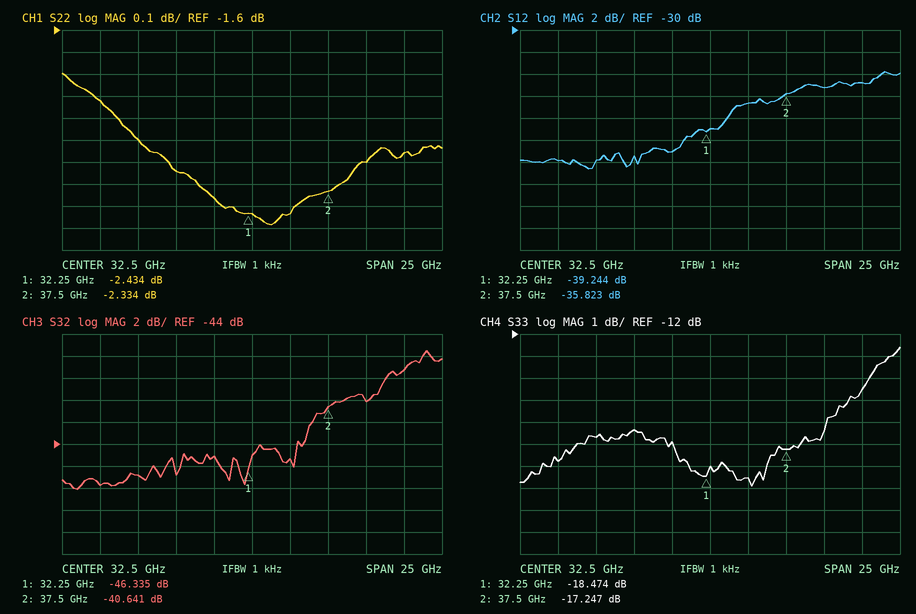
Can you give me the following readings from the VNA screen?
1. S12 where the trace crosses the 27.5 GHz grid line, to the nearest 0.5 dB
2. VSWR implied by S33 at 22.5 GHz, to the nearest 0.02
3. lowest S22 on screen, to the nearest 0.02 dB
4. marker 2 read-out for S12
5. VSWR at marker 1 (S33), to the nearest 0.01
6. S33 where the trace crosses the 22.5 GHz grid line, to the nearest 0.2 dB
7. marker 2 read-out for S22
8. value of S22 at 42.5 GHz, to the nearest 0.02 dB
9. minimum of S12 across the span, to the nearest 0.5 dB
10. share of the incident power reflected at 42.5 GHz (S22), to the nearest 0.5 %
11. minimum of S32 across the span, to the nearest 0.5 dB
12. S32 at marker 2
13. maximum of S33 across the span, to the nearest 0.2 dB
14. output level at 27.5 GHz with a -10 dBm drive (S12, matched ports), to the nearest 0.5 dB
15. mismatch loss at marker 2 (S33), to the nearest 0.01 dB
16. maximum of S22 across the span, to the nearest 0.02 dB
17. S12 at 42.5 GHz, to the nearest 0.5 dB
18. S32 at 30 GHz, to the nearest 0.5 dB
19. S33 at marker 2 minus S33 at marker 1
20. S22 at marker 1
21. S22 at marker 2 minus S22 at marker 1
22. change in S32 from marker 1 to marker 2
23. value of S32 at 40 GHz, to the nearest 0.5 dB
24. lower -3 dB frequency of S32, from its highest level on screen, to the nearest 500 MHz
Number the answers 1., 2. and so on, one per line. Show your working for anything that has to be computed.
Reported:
1. -41.5 dB
2. |Γ| = 10^(-17.8/20) = 0.1288; VSWR = (1 + 0.1288)/(1 − 0.1288) ≈ 1.30
3. -2.48 dB
4. -35.823 dB
5. (1 + 0.1192)/(1 − 0.1192) ≈ 1.27
6. -17.8 dB
7. -2.334 dB
8. -2.16 dB
9. -42.5 dB
10. 10^(-2.16/10) ≈ 60.8 %, so 61.0 % to the nearest 0.5 %
11. -48.0 dB
12. -40.641 dB
13. -12.6 dB
14. -10 dBm + (-41.5 dB) = -51.5 dBm
15. −10 log10(1 − 10^(-17.247/10)) ≈ 0.08 dB
16. -1.80 dB
17. -35.0 dB
18. -45.0 dB
19. -17.247 − (-18.474) = 1.227 dB
20. -2.434 dB
21. -2.334 − (-2.434) = 0.100 dB
22. -40.641 − (-46.335) = 5.694 dB
23. -40.0 dB
24. 41.0 GHz
